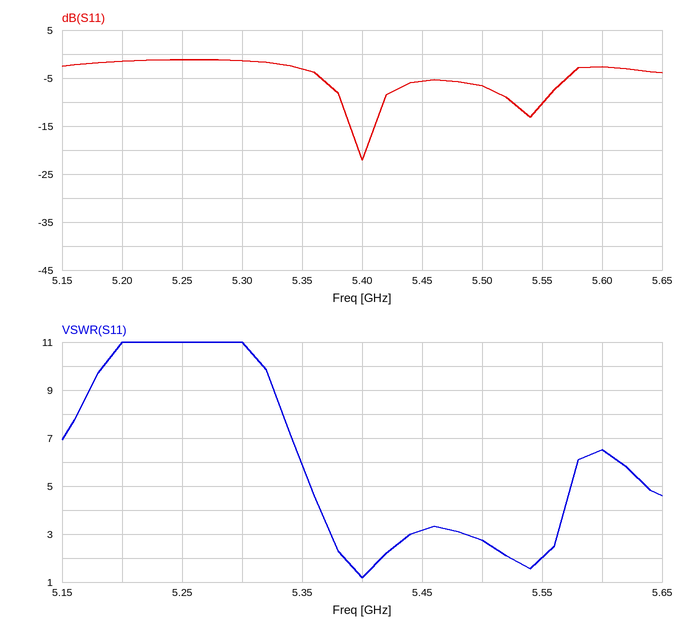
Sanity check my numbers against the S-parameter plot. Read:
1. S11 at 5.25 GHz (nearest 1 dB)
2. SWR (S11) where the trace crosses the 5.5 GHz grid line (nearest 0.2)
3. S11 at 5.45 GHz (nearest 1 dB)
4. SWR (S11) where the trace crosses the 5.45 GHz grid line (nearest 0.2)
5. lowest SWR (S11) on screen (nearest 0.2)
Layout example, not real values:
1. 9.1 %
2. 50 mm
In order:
1. -1 dB
2. 2.8
3. -6 dB
4. 3.2
5. 1.2
